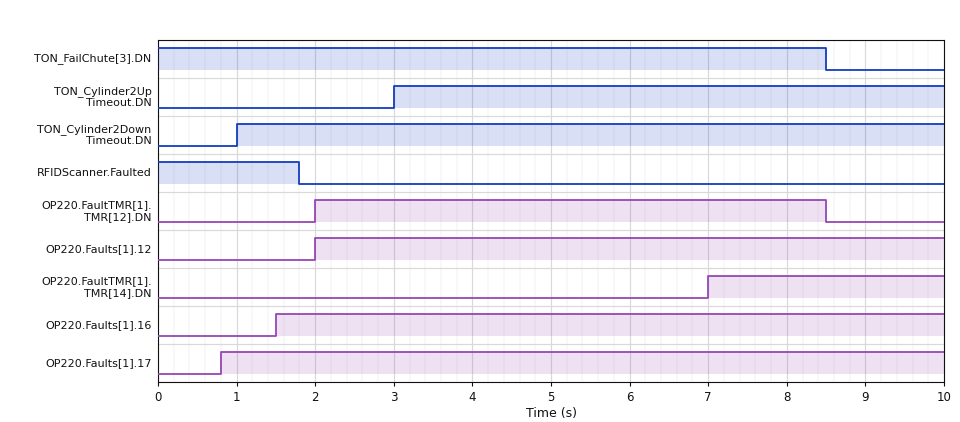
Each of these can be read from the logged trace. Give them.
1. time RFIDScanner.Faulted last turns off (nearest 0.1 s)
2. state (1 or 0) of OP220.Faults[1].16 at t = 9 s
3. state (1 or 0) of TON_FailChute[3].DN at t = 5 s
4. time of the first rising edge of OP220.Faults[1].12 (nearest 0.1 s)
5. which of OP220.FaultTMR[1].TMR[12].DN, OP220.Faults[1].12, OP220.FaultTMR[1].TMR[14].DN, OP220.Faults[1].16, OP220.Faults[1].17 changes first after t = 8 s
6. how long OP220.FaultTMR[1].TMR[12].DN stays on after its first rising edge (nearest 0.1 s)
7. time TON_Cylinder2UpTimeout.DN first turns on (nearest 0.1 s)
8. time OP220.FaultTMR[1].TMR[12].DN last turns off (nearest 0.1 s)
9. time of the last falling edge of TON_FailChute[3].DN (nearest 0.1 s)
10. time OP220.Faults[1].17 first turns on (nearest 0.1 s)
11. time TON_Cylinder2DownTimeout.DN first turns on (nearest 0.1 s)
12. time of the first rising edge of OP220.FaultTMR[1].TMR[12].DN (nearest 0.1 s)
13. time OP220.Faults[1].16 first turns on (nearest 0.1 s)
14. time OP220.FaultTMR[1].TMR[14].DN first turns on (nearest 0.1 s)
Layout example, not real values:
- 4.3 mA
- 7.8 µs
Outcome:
- 1.8 s
- 1
- 1
- 2.0 s
- OP220.FaultTMR[1].TMR[12].DN
- 6.5 s
- 3.0 s
- 8.5 s
- 8.5 s
- 0.8 s
- 1.0 s
- 2.0 s
- 1.5 s
- 7.0 s
